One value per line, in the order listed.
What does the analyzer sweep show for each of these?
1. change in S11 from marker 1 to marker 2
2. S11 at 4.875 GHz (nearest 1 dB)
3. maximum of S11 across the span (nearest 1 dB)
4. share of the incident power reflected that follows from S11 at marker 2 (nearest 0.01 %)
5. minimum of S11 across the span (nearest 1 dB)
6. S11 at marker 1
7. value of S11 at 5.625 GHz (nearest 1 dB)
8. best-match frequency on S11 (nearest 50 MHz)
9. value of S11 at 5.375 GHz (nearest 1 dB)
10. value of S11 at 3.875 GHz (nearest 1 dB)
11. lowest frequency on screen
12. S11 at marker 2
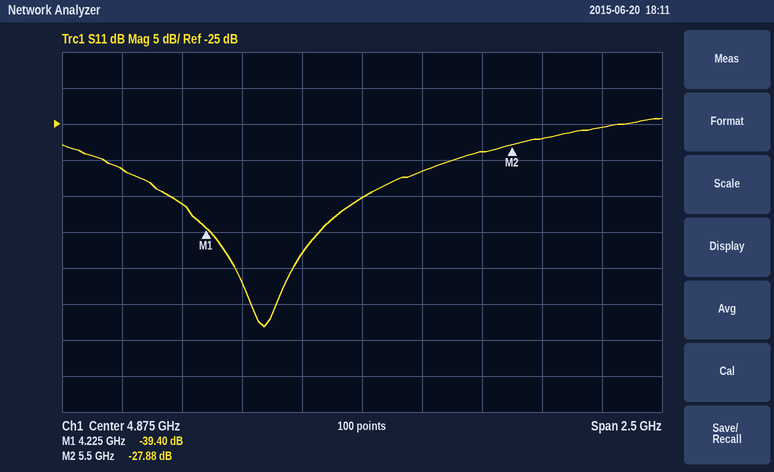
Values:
11.52 dB
-35 dB
-24 dB
0.16 %
-53 dB
-39.40 dB
-27 dB
4.45 GHz
-29 dB
-31 dB
3.625 GHz
-27.88 dB
